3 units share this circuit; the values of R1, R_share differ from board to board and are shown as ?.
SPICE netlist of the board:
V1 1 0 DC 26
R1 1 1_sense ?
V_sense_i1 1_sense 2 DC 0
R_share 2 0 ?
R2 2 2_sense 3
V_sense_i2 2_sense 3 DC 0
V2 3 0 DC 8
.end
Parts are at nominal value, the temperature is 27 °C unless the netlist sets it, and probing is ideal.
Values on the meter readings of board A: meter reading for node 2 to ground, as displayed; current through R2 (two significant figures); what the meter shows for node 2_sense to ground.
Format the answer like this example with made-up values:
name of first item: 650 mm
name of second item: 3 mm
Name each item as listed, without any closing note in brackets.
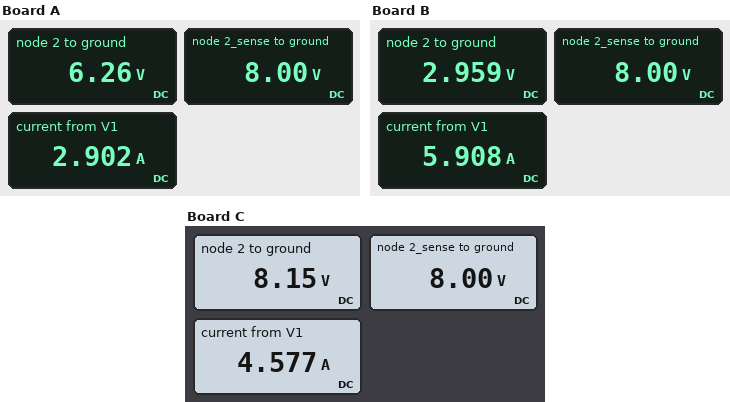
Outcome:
meter reading for node 2 to ground, as displayed: 6.26 V
current through R2: 580 mA
what the meter shows for node 2_sense to ground: 8.00 V
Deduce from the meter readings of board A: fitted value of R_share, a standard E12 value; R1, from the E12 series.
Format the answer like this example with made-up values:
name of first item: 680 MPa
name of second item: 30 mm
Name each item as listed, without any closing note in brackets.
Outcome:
fitted value of R_share, a standard E12 value: 1.8 Ω
R1, from the E12 series: 6.8 Ω
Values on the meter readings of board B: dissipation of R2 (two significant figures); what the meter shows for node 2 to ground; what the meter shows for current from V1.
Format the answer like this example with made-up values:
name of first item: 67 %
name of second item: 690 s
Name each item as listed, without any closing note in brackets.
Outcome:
dissipation of R2: 8.5 W
what the meter shows for node 2 to ground: 2.959 V
what the meter shows for current from V1: 5.908 A
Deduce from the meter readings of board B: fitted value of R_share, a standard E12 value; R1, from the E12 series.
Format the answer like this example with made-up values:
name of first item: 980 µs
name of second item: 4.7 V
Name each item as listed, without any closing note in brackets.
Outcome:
fitted value of R_share, a standard E12 value: 0.39 Ω
R1, from the E12 series: 3.9 Ω
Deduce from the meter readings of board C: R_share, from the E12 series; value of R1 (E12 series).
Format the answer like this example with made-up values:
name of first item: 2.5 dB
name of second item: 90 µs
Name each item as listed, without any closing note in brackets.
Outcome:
R_share, from the E12 series: 1.8 Ω
value of R1: 3.9 Ω
